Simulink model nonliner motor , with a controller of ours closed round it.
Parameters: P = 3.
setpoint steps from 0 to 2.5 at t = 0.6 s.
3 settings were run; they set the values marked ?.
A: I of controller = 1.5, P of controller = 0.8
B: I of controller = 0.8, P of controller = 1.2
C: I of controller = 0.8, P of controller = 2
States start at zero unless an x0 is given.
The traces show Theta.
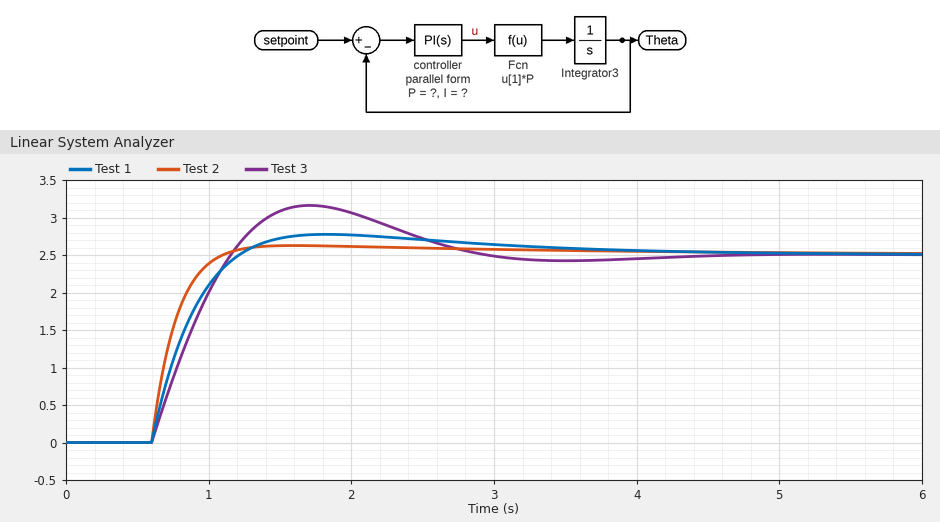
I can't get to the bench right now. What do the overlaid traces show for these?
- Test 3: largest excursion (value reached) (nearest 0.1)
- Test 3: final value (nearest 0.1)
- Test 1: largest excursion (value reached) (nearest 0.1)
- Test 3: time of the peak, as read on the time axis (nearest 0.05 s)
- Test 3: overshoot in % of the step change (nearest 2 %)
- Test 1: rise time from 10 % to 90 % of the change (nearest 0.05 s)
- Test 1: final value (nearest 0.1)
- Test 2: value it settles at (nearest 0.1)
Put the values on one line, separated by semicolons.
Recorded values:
3.2; 2.5; 2.8; 1.70 s; 26 %; 0.45 s; 2.5; 2.5
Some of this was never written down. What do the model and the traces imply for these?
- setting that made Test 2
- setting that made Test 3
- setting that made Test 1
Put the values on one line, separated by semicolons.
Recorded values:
C; A; B
